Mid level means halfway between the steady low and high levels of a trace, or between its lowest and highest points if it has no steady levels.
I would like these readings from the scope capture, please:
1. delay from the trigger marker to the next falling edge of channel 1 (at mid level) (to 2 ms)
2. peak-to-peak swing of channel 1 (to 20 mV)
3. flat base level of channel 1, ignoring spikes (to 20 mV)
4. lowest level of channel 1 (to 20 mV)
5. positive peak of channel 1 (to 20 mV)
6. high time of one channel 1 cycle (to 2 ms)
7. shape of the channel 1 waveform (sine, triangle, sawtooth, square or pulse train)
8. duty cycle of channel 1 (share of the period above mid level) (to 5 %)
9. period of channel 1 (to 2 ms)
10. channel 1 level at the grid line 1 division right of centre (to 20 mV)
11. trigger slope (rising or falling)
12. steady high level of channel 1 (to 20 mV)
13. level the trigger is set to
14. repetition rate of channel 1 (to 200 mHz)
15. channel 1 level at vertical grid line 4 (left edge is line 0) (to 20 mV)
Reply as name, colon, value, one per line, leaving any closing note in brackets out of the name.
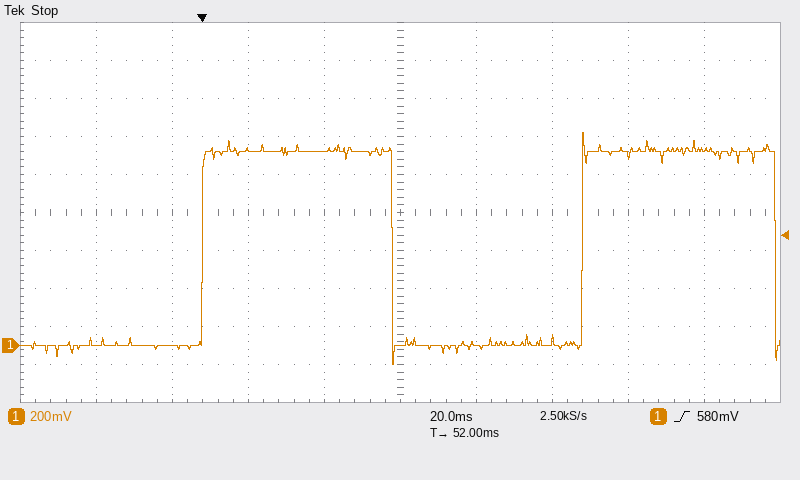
delay from the trigger marker to the next falling edge of channel 1 (at mid level): 50 ms
peak-to-peak swing of channel 1: 1.22 V
flat base level of channel 1, ignoring spikes: 0 mV
lowest level of channel 1: -100 mV
positive peak of channel 1: 1.12 V
high time of one channel 1 cycle: 50 ms
shape of the channel 1 waveform: square
duty cycle of channel 1 (share of the period above mid level): 50 %
period of channel 1: 100 ms
channel 1 level at the grid line 1 division right of centre: 0 mV
trigger slope: rising
steady high level of channel 1: 1.02 V
level the trigger is set to: 580 mV
repetition rate of channel 1: 10.0 Hz
channel 1 level at vertical grid line 4 (left edge is line 0): 1.02 V
